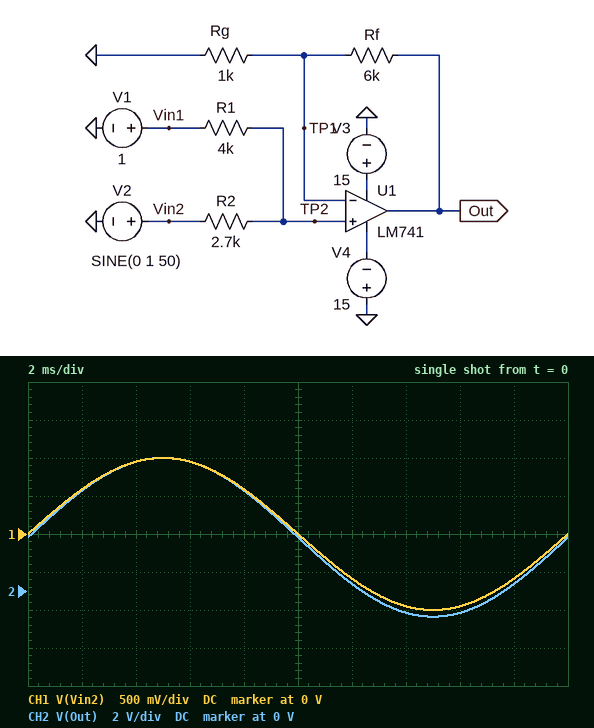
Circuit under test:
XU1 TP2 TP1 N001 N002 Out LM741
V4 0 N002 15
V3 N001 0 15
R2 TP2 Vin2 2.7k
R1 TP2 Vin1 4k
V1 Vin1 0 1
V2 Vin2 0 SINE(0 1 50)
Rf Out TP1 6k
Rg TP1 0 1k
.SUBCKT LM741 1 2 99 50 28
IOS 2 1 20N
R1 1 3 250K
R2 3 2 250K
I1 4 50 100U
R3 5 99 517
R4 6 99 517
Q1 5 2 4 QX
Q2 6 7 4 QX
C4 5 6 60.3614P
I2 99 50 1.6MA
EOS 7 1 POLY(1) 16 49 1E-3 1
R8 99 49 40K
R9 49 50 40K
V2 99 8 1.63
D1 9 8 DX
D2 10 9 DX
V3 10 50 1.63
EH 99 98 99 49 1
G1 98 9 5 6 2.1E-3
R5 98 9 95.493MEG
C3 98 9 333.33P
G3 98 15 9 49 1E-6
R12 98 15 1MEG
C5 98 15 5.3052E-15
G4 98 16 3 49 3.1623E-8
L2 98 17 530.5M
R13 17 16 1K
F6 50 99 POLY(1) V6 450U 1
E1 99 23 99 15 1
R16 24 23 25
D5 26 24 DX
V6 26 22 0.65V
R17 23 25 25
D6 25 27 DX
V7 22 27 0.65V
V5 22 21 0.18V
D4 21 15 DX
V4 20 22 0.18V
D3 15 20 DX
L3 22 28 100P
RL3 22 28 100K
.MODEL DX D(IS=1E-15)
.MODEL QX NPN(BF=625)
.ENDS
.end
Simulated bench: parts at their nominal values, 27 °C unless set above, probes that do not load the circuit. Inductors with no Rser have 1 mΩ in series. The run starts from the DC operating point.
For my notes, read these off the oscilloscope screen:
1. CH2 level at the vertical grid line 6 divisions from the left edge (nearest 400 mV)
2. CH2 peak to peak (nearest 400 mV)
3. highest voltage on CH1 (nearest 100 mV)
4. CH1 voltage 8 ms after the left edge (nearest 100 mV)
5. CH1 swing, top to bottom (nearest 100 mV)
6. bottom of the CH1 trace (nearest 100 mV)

400 mV
8.4 V
1.0 V
600 mV
2.0 V
-1.0 V
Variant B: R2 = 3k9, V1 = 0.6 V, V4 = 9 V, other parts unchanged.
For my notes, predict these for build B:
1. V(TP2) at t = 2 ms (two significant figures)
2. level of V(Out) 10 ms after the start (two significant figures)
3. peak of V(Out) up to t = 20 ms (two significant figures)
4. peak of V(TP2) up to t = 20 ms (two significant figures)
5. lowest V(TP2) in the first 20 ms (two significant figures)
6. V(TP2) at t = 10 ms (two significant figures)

590 mV
2.1 V
5.6 V
800 mV
-210 mV
300 mV
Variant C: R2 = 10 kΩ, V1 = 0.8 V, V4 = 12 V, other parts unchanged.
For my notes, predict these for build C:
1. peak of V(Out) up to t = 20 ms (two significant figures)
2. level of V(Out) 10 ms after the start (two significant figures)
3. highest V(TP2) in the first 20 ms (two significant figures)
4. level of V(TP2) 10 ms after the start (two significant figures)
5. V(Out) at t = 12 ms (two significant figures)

6.0 V
4.0 V
860 mV
570 mV
2.8 V
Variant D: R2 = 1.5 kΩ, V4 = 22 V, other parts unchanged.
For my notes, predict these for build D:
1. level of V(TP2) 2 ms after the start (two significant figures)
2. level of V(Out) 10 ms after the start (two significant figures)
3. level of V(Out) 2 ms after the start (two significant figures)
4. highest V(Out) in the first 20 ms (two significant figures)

700 mV
1.9 V
4.9 V
7.0 V
